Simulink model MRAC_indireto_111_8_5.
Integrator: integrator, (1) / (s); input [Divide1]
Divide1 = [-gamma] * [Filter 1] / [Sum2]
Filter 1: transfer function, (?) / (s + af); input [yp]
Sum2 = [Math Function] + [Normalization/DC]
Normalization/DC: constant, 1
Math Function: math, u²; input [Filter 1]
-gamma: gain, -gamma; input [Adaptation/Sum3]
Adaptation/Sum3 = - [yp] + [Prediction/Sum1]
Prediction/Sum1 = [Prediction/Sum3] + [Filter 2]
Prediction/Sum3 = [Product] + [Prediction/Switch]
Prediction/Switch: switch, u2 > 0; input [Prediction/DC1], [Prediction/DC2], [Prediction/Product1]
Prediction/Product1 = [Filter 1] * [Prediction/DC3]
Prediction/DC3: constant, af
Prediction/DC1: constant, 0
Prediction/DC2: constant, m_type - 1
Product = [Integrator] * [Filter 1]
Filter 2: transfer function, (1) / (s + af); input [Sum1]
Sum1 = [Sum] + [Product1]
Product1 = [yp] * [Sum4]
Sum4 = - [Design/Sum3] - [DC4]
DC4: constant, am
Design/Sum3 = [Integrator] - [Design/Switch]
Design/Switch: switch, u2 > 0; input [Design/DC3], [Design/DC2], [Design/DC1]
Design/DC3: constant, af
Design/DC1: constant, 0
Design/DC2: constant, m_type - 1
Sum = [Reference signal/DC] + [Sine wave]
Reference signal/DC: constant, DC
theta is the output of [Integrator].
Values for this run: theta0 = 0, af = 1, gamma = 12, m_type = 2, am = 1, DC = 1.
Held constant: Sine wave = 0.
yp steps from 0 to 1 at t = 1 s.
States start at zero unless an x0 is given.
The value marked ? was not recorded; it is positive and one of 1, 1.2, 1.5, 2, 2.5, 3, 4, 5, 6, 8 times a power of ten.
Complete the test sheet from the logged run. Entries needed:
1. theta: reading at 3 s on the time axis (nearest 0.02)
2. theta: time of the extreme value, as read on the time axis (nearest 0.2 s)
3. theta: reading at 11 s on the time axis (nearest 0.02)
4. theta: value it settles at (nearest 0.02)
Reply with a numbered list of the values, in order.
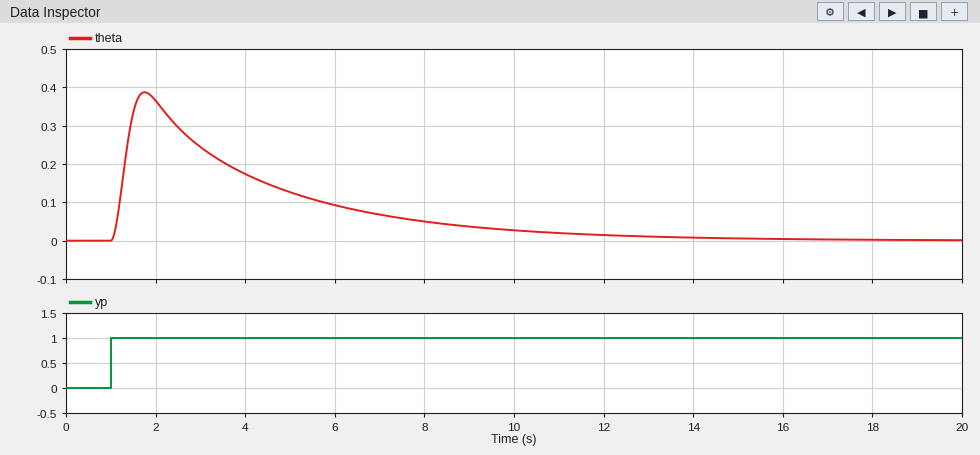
1. 0.24
2. 1.8 s
3. 0.02
4. 0.00
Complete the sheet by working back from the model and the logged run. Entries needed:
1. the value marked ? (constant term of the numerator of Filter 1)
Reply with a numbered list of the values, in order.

1. 1.5
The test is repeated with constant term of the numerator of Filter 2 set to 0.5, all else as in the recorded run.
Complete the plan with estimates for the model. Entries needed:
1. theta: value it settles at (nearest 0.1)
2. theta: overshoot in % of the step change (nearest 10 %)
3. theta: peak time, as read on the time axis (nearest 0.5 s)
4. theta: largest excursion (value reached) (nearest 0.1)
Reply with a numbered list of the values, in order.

1. 0.5
2. 80 %
3. 2.0 s
4. 0.9
